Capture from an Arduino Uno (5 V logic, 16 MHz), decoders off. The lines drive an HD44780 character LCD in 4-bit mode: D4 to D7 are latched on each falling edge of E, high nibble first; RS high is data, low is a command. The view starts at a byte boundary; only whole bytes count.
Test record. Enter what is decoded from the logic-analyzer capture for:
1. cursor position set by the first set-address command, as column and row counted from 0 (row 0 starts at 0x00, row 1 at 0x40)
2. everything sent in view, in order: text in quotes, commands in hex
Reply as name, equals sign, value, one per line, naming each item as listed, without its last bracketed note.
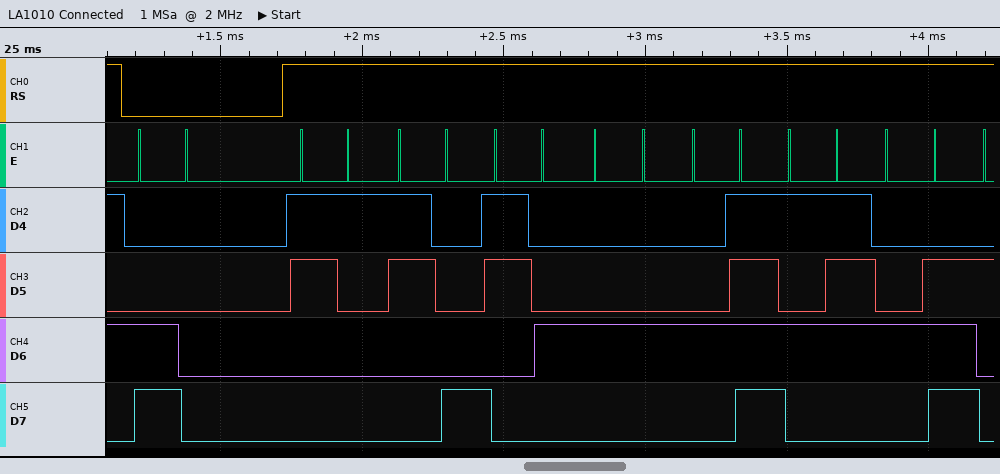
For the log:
cursor position set by the first set-address command, as column and row counted from 0 = column 0, row 1
everything sent in view, in order: text in quotes, commands in hex = 0xC0 "184DOWN"
